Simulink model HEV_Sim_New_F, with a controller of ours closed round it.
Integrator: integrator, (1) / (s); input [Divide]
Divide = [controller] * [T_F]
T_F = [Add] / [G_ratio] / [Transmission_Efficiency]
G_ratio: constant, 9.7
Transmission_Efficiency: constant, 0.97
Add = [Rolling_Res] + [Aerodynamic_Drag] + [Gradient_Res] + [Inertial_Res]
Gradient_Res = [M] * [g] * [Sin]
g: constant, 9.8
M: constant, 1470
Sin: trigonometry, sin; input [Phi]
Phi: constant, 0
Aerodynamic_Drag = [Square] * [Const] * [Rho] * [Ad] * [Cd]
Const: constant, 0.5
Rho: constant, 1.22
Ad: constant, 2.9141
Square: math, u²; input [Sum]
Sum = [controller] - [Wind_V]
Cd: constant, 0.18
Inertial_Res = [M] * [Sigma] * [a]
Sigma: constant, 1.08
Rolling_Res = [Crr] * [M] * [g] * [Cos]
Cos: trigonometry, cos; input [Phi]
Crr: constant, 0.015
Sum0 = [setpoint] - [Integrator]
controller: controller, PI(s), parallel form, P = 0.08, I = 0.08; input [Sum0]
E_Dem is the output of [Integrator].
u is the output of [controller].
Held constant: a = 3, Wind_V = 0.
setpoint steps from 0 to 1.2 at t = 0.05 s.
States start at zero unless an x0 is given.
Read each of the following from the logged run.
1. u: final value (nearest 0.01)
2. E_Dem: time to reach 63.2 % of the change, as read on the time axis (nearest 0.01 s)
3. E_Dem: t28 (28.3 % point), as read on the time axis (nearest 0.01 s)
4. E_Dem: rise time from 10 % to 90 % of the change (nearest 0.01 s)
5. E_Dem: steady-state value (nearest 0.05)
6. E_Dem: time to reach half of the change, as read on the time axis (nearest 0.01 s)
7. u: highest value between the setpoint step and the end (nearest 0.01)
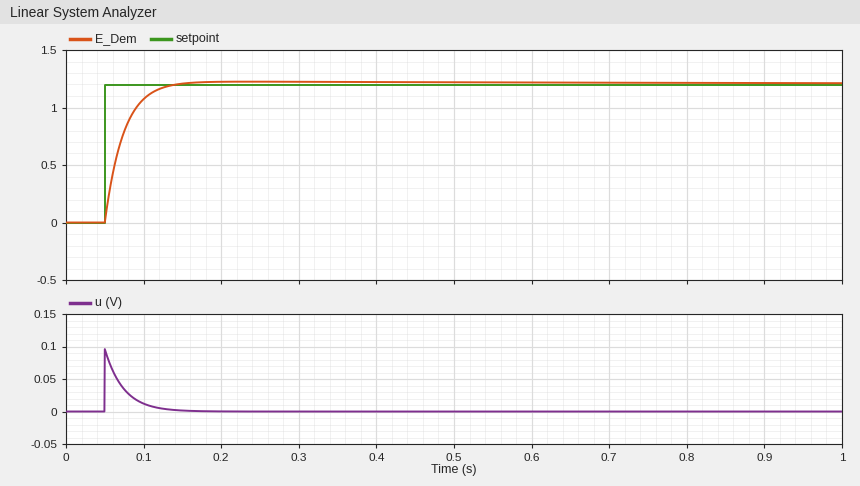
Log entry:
0.00
0.07 s
0.06 s
0.05 s
1.20
0.07 s
0.10
